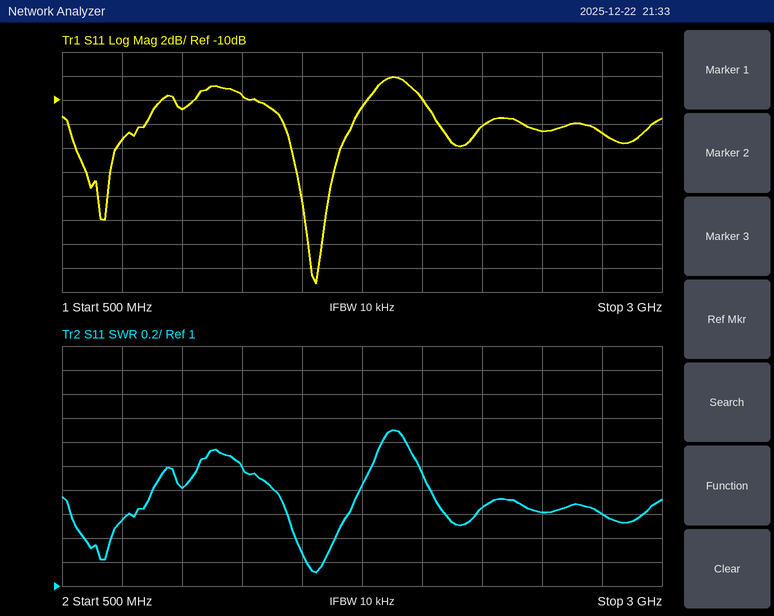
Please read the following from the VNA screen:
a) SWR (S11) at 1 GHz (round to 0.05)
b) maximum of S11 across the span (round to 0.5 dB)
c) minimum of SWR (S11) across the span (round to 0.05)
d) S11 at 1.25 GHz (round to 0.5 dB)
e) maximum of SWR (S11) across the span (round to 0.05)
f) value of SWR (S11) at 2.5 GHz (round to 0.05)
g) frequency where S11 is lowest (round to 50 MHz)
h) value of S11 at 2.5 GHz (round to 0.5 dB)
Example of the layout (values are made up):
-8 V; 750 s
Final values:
1.80; -8.0 dB; 1.10; -9.5 dB; 2.30; 1.60; 1.55 GHz; -12.5 dB
